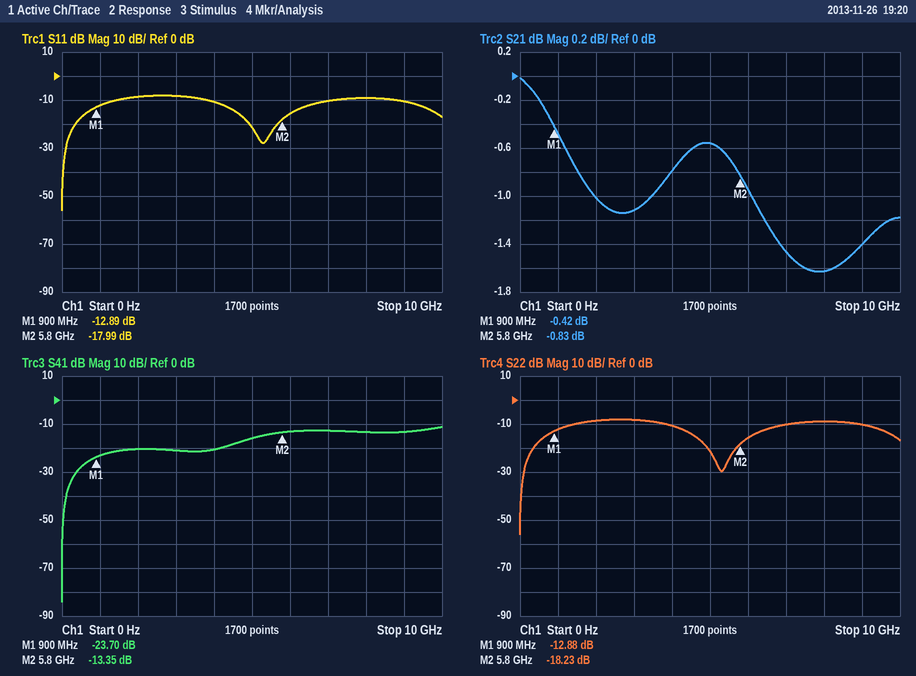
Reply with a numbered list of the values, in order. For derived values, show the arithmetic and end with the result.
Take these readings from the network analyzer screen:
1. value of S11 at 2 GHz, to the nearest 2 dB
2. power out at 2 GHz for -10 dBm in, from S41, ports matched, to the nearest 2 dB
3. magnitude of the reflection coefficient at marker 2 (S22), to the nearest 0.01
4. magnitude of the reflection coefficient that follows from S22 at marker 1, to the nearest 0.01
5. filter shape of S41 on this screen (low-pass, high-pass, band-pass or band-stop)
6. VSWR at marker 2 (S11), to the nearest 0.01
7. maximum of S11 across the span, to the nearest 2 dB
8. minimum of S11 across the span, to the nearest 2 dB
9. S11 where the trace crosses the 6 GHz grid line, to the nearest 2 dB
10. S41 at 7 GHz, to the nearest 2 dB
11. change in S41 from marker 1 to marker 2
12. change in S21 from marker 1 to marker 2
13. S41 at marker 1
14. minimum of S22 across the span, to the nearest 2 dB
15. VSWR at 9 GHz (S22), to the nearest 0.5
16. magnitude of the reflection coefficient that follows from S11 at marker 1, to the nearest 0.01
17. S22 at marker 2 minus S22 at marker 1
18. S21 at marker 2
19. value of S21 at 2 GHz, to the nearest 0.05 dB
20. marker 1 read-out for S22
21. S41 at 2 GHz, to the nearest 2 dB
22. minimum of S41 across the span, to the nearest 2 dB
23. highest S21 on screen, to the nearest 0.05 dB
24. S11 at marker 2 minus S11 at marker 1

1. -8 dB
2. -10 dBm + (-20 dB) = -30 dBm
3. 10^(-18.23/20) ≈ 0.12
4. 10^(-12.88/20) ≈ 0.23
5. high-pass
6. (1 + 0.1260)/(1 − 0.1260) ≈ 1.29
7. -8 dB
8. -56 dB
9. -16 dB
10. -12 dB
11. -13.35 − (-23.7) = 10.35 dB
12. -0.83 − (-0.42) = -0.41 dB
13. -23.70 dB
14. -56 dB
15. |Γ| = 10^(-10/20) = 0.3162; VSWR = (1 + 0.3162)/(1 − 0.3162) ≈ 1.92, so 2.0 to the nearest 0.5
16. 10^(-12.89/20) ≈ 0.23
17. -18.23 − (-12.88) = -5.35 dB
18. -0.83 dB
19. -1.00 dB
20. -12.88 dB
21. -20 dB
22. -84 dB
23. 0.00 dB
24. -17.99 − (-12.89) = -5.10 dB
